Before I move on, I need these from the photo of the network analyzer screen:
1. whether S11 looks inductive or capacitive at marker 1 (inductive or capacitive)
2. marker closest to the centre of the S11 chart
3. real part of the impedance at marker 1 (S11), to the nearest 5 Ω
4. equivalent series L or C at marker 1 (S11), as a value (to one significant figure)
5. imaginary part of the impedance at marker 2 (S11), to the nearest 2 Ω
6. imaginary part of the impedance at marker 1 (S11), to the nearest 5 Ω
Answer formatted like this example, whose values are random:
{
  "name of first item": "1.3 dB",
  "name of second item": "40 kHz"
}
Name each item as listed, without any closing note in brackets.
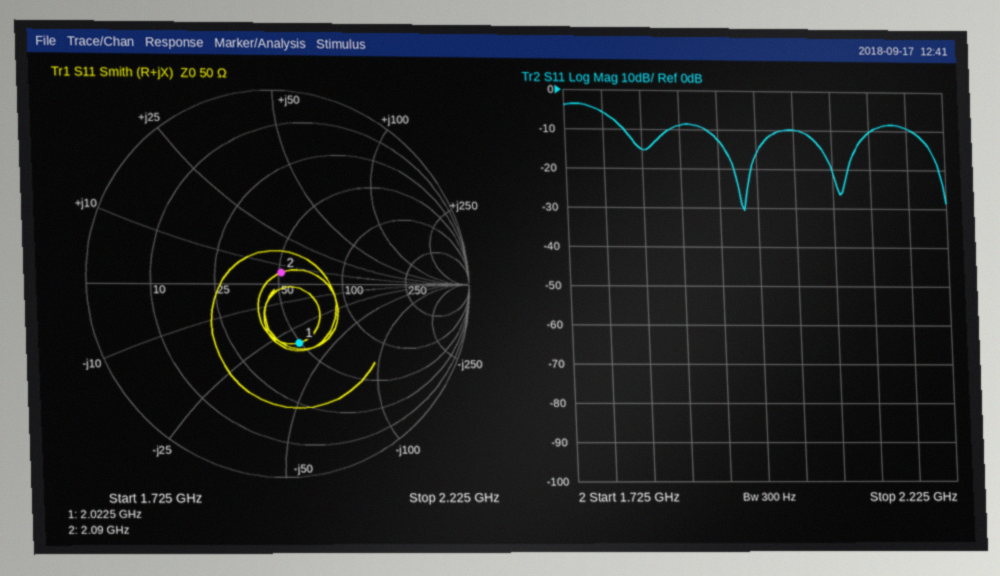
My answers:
{
  "whether S11 looks inductive or capacitive at marker 1": "capacitive",
  "marker closest to the centre of the S11 chart": "marker 2",
  "real part of the impedance at marker 1 (S11), to the nearest 5 Ω": "50 Ω",
  "equivalent series L or C at marker 1 (S11), as a value": "2 pF",
  "imaginary part of the impedance at marker 2 (S11), to the nearest 2 Ω": "+6 Ω",
  "imaginary part of the impedance at marker 1 (S11), to the nearest 5 Ω": "-35 Ω"
}
